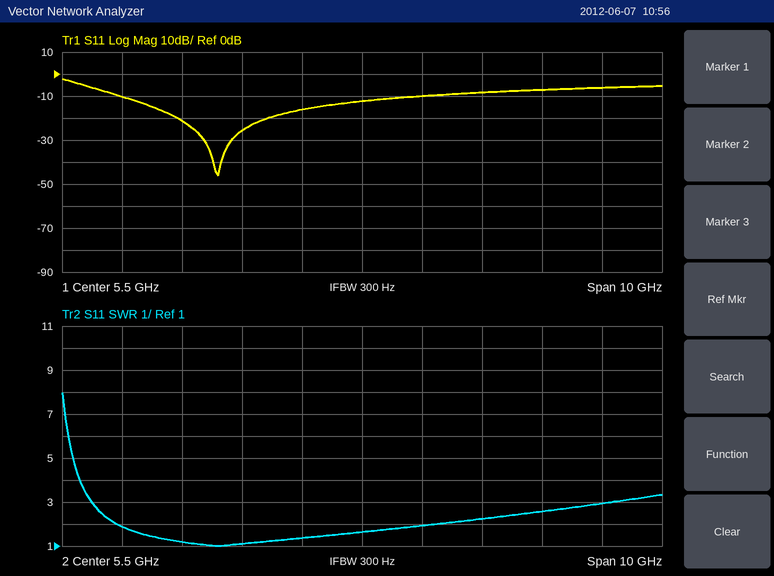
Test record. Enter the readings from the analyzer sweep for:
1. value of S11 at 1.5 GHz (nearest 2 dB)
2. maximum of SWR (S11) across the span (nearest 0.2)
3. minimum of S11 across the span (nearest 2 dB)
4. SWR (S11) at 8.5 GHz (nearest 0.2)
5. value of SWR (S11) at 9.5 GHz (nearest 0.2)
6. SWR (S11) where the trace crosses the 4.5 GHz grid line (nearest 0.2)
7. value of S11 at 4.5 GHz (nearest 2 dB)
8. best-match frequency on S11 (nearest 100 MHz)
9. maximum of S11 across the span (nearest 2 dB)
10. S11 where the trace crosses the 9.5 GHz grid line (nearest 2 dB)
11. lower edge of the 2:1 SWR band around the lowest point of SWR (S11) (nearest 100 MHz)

-10 dB
8.0
-46 dB
2.6
3.0
1.4
-16 dB
3.1 GHz
-2 dB
-6 dB
1.4 GHz
